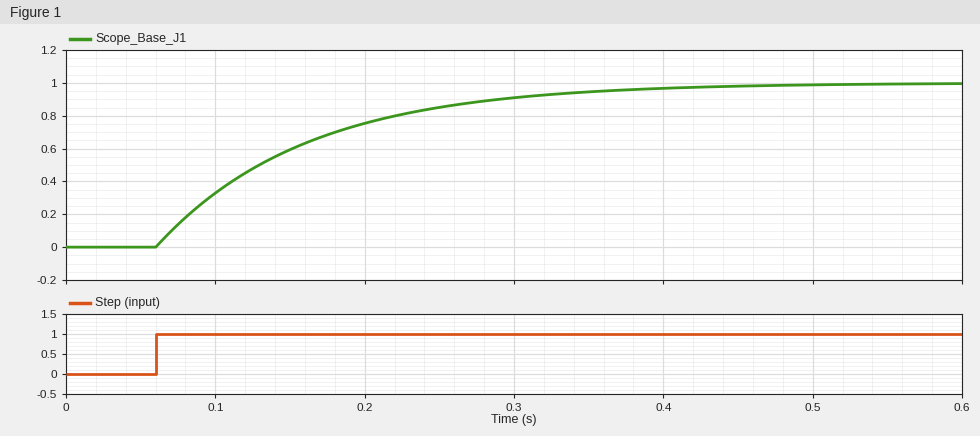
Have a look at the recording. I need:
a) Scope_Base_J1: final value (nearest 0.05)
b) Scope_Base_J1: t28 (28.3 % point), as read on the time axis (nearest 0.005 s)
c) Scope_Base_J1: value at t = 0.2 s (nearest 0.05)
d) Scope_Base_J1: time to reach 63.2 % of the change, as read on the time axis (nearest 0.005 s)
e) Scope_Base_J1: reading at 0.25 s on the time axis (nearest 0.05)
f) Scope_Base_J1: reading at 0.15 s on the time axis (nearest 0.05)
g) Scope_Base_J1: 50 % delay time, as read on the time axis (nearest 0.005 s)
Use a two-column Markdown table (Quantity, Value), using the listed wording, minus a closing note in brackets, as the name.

| Quantity | Value |
|---|---|
| Scope_Base_J1: final value | 1.00 |
| Scope_Base_J1: t28 (28.3 % point), as read on the time axis | 0.095 s |
| Scope_Base_J1: value at t = 0.2 s | 0.75 |
| Scope_Base_J1: time to reach 63.2 % of the change, as read on the time axis | 0.160 s |
| Scope_Base_J1: reading at 0.25 s on the time axis | 0.85 |
| Scope_Base_J1: reading at 0.15 s on the time axis | 0.60 |
| Scope_Base_J1: 50 % delay time, as read on the time axis | 0.130 s |
